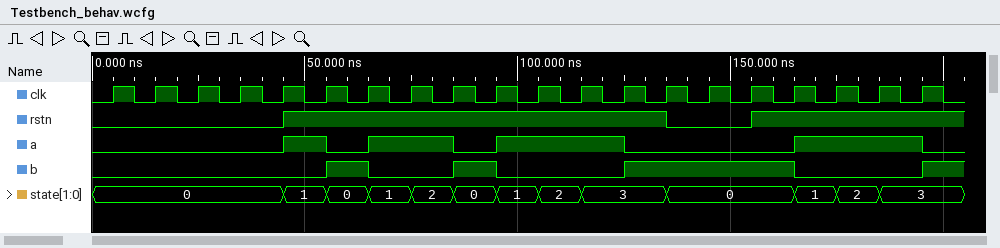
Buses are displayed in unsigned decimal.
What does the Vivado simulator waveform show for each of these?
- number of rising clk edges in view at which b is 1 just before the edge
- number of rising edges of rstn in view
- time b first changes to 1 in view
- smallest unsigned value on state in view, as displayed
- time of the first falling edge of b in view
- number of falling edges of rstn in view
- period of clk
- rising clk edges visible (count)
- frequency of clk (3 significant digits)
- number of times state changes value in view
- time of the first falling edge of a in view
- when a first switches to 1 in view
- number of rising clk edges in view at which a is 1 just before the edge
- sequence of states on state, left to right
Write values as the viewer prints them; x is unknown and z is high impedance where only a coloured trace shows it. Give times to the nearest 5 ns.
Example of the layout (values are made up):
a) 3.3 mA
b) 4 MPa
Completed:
a) 6
b) 2
c) 55 ns
d) 0
e) 65 ns
f) 1
g) 10 ns
h) 20
i) 100 MHz
j) 12
k) 55 ns
l) 45 ns
m) 9
n) 0, 1, 0, 1, 2, 0, 1, 2, 3, 0, 1, 2, 3
